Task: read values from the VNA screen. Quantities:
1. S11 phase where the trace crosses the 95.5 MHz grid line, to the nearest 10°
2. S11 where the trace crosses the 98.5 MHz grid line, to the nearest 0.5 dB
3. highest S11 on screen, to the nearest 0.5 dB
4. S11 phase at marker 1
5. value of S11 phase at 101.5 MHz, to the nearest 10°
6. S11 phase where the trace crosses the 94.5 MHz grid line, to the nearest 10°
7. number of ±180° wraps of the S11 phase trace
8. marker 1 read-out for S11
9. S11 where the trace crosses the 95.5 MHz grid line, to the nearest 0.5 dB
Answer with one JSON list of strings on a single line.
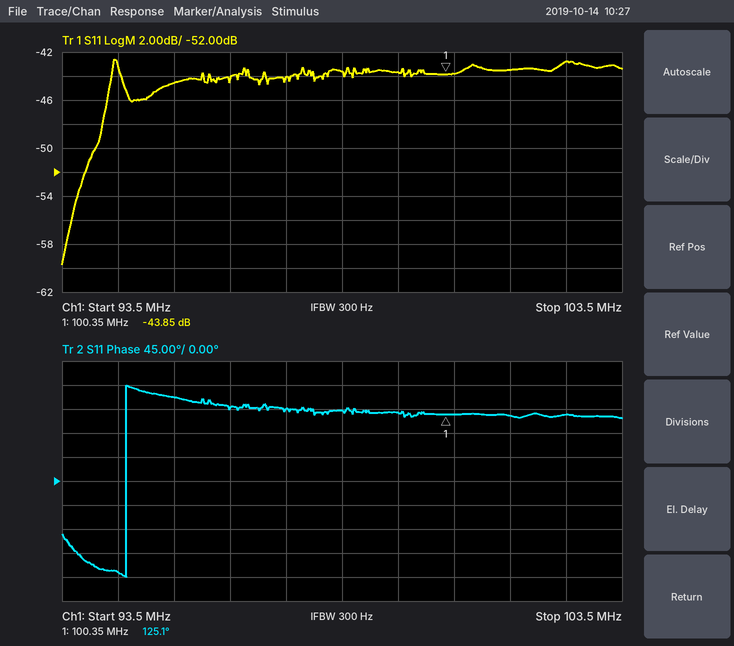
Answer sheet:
["160°", "-43.5 dB", "-42.5 dB", "125.1°", "120°", "-170°", "1", "-43.85 dB", "-44.5 dB"]
